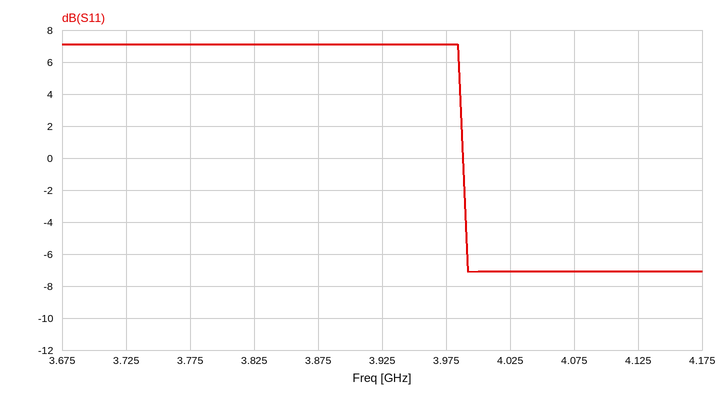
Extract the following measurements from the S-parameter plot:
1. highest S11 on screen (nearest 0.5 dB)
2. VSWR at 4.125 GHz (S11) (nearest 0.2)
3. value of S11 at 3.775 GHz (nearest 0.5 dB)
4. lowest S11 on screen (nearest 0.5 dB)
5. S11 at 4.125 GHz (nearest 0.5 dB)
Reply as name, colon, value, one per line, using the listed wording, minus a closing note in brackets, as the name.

highest S11 on screen: 7.0 dB
VSWR at 4.125 GHz (S11): 2.6
value of S11 at 3.775 GHz: 7.0 dB
lowest S11 on screen: -7.0 dB
S11 at 4.125 GHz: -7.0 dB
